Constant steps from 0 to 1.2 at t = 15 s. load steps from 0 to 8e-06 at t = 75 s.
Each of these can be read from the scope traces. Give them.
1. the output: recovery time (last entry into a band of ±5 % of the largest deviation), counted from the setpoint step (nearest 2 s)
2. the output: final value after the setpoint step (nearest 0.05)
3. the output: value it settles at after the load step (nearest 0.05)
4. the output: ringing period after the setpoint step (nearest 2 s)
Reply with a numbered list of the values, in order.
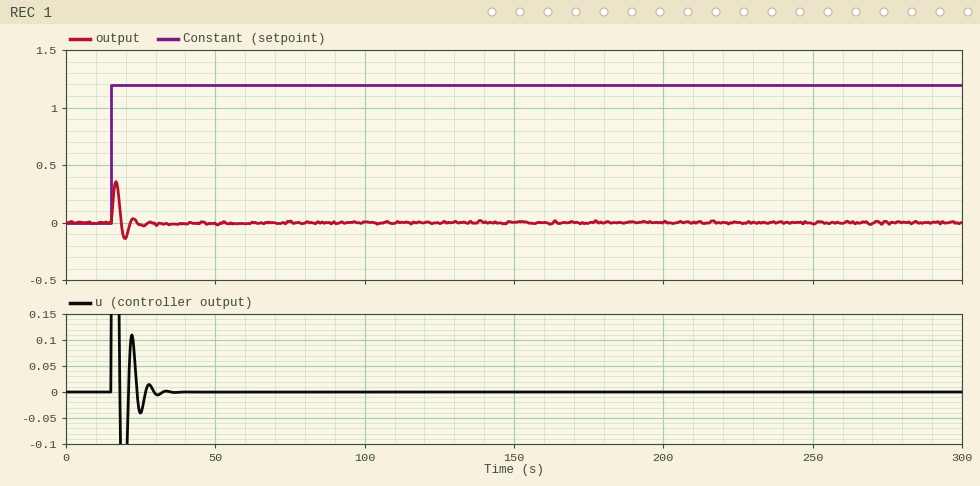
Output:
1. 12 s
2. 0.00
3. 0.00
4. 6 s
